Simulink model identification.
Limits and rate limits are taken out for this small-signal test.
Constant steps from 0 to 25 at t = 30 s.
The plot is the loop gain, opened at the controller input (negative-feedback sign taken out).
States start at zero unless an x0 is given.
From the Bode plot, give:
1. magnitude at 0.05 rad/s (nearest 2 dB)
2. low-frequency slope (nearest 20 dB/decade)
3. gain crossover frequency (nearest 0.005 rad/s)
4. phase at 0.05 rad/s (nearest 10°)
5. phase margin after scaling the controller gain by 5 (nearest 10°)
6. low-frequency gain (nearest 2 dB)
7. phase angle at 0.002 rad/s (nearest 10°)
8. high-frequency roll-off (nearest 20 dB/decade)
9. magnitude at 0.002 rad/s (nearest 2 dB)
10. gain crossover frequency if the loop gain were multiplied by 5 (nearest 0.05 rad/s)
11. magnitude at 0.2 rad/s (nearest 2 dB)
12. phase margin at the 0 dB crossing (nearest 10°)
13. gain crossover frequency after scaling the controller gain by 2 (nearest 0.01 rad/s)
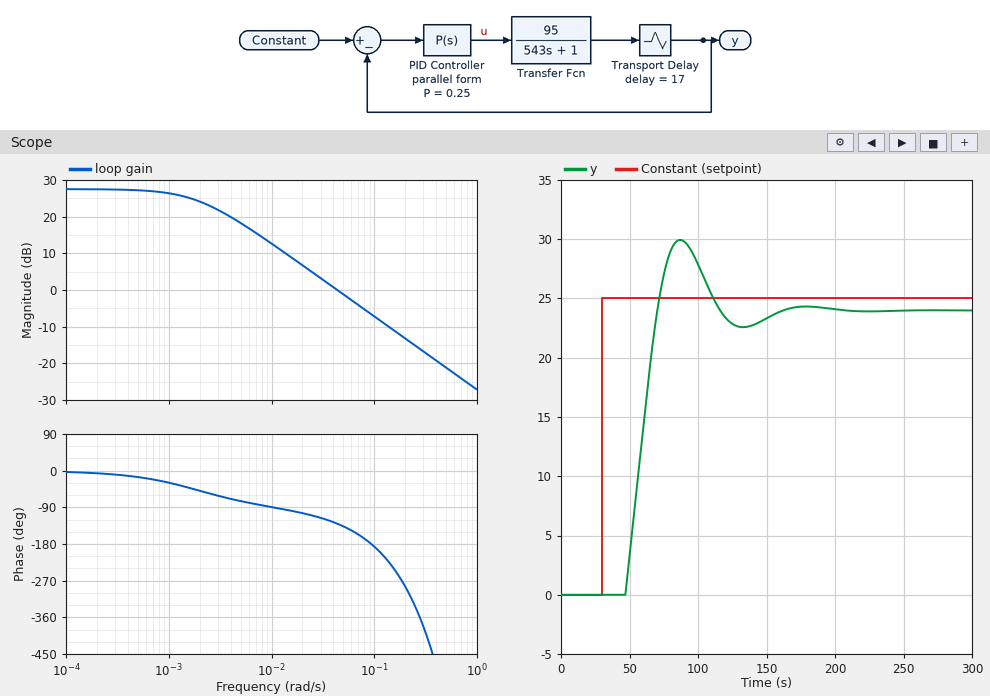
-2 dB
0 dB/decade
0.045 rad/s
-140°
-120°
28 dB
-50°
-20 dB/decade
24 dB
0.20 rad/s
-14 dB
50°
0.09 rad/s
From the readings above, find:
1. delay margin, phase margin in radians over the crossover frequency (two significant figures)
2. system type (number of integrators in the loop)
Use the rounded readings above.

19 s
0
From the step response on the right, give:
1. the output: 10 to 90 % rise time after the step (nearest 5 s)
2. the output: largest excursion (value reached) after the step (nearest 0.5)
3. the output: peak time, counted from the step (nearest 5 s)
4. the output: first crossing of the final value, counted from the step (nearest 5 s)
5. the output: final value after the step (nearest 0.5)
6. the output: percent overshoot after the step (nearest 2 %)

20 s
30.0
55 s
40 s
24.0
24 %
